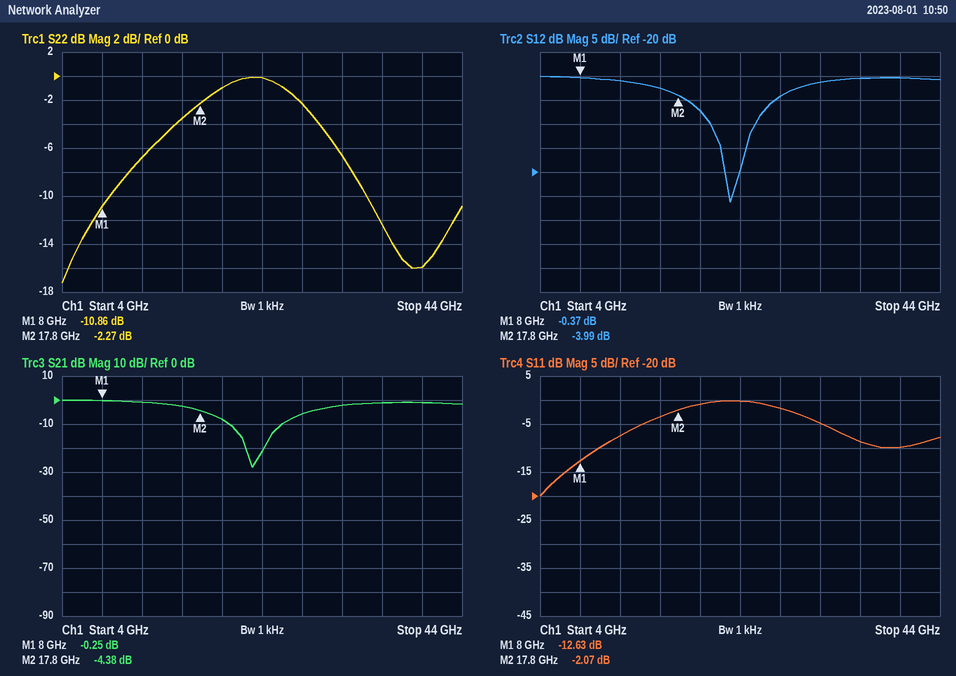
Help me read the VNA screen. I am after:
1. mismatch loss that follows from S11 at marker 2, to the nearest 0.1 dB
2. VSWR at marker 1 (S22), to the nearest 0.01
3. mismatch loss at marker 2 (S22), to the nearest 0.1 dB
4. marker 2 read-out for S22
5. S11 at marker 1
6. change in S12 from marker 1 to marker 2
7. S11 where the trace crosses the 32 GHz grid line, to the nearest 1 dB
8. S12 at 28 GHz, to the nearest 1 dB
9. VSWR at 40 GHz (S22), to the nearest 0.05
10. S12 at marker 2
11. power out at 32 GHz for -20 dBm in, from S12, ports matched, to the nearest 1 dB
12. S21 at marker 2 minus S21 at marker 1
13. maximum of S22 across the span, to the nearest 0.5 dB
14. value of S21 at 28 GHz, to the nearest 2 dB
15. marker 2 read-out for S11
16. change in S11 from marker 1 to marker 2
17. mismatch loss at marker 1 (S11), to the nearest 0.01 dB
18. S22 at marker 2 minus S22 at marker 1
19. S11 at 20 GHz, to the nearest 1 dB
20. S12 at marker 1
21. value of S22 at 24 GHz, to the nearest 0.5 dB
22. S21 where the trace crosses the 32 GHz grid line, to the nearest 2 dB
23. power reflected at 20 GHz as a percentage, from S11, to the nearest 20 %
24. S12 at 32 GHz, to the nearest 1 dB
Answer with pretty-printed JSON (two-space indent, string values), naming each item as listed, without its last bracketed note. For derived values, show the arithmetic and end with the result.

{
  "mismatch loss that follows from S11 at marker 2, to the nearest 0.1 dB": "−10 log10(1 − 10^(-2.07/10)) ≈ 4.2 dB",
  "VSWR at marker 1 (S22), to the nearest 0.01": "(1 + 0.2864)/(1 − 0.2864) ≈ 1.80",
  "mismatch loss at marker 2 (S22), to the nearest 0.1 dB": "−10 log10(1 − 10^(-2.27/10)) ≈ 3.9 dB",
  "marker 2 read-out for S22": "-2.27 dB",
  "S11 at marker 1": "-12.63 dB",
  "change in S12 from marker 1 to marker 2": "-3.99 − (-0.37) = -3.62 dB",
  "S11 where the trace crosses the 32 GHz grid line, to the nearest 1 dB": "-5 dB",
  "S12 at 28 GHz, to the nearest 1 dB": "-4 dB",
  "VSWR at 40 GHz (S22), to the nearest 0.05": "|Γ| = 10^(-16/20) = 0.1585; VSWR = (1 + 0.1585)/(1 − 0.1585) ≈ 1.38, so 1.40 to the nearest 0.05",
  "S12 at marker 2": "-3.99 dB",
  "power out at 32 GHz for -20 dBm in, from S12, ports matched, to the nearest 1 dB": "-20 dBm + (-1 dB) = -21 dBm",
  "S21 at marker 2 minus S21 at marker 1": "-4.38 − (-0.25) = -4.13 dB",
  "maximum of S22 across the span, to the nearest 0.5 dB": "0.0 dB",
  "value of S21 at 28 GHz, to the nearest 2 dB": "-6 dB",
  "marker 2 read-out for S11": "-2.07 dB",
  "change in S11 from marker 1 to marker 2": "-2.07 − (-12.63) = 10.56 dB",
  "mismatch loss at marker 1 (S11), to the nearest 0.01 dB": "−10 log10(1 − 10^(-12.63/10)) ≈ 0.24 dB",
  "S22 at marker 2 minus S22 at marker 1": "-2.27 − (-10.86) = 8.59 dB",
  "S11 at 20 GHz, to the nearest 1 dB": "-1 dB",
  "S12 at marker 1": "-0.37 dB",
  "value of S22 at 24 GHz, to the nearest 0.5 dB": "0.0 dB",
  "S21 where the trace crosses the 32 GHz grid line, to the nearest 2 dB": "-2 dB",
  "power reflected at 20 GHz as a percentage, from S11, to the nearest 20 %": "10^(-1/10) ≈ 79.4 %, so 80 % to the nearest 20 %",
  "S12 at 32 GHz, to the nearest 1 dB": "-1 dB"
}
